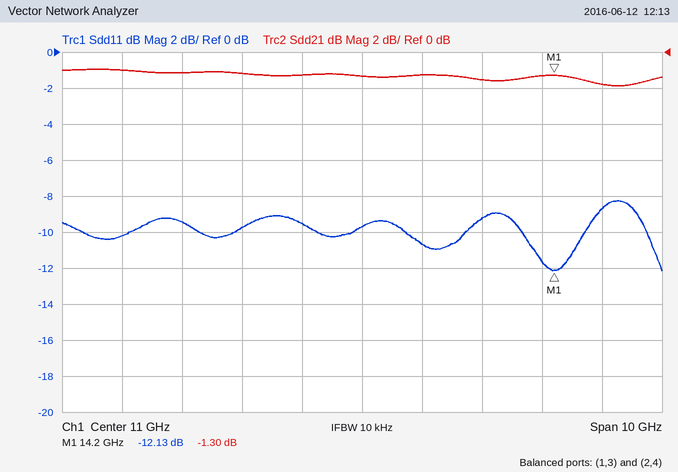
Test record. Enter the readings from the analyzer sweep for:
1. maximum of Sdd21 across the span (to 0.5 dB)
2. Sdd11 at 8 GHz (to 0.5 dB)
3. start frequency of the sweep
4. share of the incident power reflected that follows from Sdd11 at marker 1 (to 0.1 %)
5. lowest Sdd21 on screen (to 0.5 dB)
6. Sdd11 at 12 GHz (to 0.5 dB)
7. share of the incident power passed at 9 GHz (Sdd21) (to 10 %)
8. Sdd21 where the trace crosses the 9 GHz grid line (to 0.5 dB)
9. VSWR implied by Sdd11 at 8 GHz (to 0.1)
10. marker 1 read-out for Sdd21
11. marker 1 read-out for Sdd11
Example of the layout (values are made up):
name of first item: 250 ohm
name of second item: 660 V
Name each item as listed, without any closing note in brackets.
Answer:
maximum of Sdd21 across the span: -1.0 dB
Sdd11 at 8 GHz: -9.5 dB
start frequency of the sweep: 6 GHz
share of the incident power reflected that follows from Sdd11 at marker 1: 6.1 %
lowest Sdd21 on screen: -2.0 dB
Sdd11 at 12 GHz: -10.5 dB
share of the incident power passed at 9 GHz (Sdd21): 80 %
Sdd21 where the trace crosses the 9 GHz grid line: -1.0 dB
VSWR implied by Sdd11 at 8 GHz: 2.0
marker 1 read-out for Sdd21: -1.30 dB
marker 1 read-out for Sdd11: -12.13 dB
